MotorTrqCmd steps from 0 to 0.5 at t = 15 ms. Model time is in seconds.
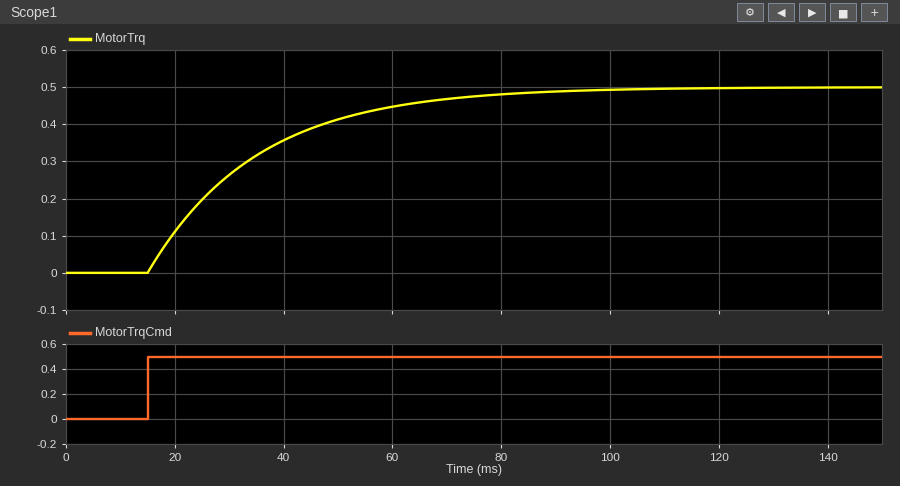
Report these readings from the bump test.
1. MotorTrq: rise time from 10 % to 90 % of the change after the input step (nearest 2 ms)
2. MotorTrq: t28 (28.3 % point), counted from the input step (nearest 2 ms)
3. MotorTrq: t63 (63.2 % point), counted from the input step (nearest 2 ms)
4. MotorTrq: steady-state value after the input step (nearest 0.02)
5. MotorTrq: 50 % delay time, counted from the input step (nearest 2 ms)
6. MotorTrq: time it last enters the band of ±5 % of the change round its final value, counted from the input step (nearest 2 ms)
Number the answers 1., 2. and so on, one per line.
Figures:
1. 44 ms
2. 6 ms
3. 20 ms
4. 0.50
5. 14 ms
6. 60 ms
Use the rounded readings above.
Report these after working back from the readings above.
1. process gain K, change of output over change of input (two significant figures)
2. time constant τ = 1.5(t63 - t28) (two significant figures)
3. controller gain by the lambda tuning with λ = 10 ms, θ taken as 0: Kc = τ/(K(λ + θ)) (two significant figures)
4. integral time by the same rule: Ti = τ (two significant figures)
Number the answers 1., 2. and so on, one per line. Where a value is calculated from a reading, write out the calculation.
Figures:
1. (0.5 - 0) / 0.5 = 1.0
2. 1.5 × (20 - 6) = 21 ms
3. 21 / (1 × (10 + 0)) = 2.1
4. 21 ms
